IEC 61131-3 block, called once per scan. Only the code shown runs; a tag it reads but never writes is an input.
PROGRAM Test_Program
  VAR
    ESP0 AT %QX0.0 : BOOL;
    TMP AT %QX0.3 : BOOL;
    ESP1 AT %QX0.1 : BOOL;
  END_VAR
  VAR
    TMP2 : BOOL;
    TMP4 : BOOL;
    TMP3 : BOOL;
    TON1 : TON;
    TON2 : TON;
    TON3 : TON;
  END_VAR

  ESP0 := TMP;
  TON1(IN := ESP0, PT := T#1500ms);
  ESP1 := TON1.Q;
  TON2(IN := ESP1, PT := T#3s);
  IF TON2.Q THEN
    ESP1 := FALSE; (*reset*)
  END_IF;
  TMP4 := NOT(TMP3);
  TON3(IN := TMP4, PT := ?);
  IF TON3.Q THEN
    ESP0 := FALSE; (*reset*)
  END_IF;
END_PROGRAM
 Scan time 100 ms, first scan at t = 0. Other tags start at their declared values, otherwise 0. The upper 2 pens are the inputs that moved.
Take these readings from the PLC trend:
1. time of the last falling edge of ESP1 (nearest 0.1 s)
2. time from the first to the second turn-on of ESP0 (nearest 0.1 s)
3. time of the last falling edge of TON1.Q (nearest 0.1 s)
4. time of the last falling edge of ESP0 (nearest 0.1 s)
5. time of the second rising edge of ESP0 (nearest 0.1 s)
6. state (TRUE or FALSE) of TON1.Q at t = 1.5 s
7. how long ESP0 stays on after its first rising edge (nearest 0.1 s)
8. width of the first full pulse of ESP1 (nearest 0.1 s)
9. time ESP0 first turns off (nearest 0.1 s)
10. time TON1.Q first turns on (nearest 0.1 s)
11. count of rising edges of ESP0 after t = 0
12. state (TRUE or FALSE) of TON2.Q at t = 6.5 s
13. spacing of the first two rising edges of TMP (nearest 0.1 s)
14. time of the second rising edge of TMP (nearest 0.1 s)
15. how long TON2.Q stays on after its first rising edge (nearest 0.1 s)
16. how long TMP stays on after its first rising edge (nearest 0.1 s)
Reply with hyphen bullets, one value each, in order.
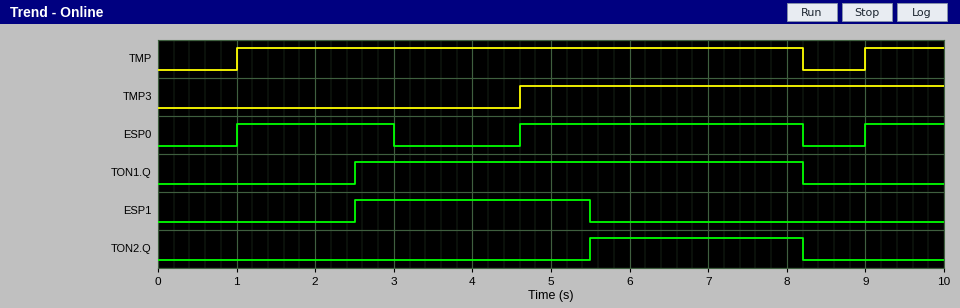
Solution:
- 5.5 s
- 3.6 s
- 8.2 s
- 8.2 s
- 4.6 s
- FALSE
- 2.0 s
- 3.0 s
- 3.0 s
- 2.5 s
- 3
- TRUE
- 8.0 s
- 9.0 s
- 2.7 s
- 7.2 s
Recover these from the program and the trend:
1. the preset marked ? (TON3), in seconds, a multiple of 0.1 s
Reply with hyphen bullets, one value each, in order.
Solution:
- 3.0 s
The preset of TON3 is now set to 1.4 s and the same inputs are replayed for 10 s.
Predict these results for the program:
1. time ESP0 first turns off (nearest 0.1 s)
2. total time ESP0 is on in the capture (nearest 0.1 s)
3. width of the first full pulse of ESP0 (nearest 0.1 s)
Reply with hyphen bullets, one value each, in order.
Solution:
- 1.4 s
- 5.0 s
- 0.4 s
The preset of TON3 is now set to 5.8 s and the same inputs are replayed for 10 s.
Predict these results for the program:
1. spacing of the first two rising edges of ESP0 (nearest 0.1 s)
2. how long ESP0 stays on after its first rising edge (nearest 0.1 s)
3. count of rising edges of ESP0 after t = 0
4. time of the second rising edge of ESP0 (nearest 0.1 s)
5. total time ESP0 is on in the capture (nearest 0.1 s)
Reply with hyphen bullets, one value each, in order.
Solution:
- 8.0 s
- 7.2 s
- 2
- 9.0 s
- 8.2 s
